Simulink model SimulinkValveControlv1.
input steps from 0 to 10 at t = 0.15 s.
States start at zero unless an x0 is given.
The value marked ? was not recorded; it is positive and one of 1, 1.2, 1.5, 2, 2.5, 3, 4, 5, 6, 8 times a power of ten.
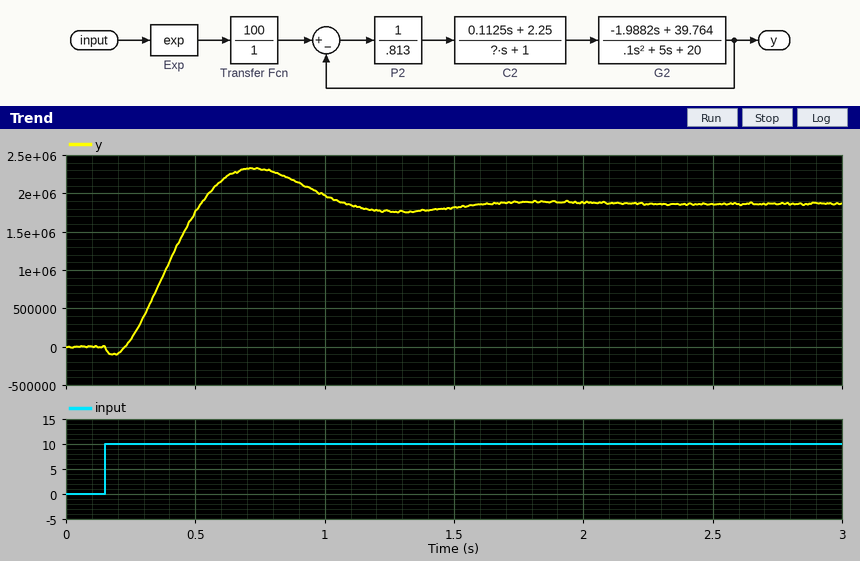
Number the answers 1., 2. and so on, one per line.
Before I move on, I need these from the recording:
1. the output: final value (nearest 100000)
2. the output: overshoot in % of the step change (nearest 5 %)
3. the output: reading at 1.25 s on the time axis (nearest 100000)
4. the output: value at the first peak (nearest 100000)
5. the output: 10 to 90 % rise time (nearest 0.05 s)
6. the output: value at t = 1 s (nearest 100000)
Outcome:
1. 1900000
2. 25 %
3. 1800000
4. 2300000
5. 0.20 s
6. 2000000
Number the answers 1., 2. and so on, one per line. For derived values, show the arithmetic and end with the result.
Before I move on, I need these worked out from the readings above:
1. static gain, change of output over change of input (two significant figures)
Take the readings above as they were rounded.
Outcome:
1. (1.9e+06 - 0) / (10 - 0) = 190000
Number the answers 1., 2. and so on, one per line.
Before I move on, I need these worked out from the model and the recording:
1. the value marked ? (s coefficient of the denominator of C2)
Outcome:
1. 0.8
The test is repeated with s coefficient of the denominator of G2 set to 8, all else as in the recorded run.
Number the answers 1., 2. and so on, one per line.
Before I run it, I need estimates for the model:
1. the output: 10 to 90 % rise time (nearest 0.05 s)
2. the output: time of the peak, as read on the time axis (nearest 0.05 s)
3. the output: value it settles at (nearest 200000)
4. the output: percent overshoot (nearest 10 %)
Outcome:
1. 0.30 s
2. 0.90 s
3. 1800000
4. 30 %
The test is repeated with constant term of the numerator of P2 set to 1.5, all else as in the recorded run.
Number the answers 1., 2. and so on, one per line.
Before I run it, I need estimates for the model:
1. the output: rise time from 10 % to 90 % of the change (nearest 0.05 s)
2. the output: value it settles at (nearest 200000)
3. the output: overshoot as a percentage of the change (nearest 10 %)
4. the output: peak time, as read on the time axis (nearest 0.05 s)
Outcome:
1. 0.15 s
2. 2000000
3. 40 %
4. 0.60 s
